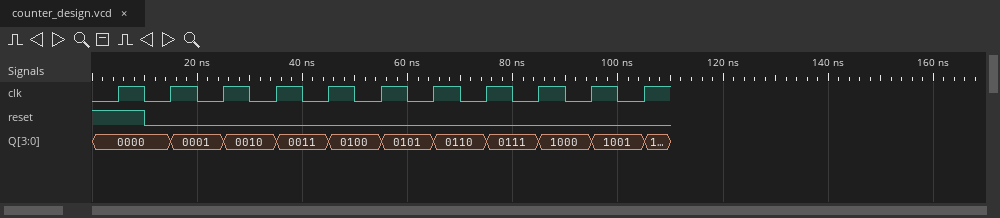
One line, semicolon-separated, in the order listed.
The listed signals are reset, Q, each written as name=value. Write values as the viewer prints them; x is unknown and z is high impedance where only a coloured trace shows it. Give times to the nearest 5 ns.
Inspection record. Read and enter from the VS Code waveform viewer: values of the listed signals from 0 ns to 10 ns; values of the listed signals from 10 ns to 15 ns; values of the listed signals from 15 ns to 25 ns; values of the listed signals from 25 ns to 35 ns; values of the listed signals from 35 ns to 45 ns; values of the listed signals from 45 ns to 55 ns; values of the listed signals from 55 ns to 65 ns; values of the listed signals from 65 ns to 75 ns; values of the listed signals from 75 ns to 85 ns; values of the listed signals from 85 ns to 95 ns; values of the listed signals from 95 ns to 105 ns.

reset=1, Q=0000; reset=0, Q=0000; reset=0, Q=0001; reset=0, Q=0010; reset=0, Q=0011; reset=0, Q=0100; reset=0, Q=0101; reset=0, Q=0110; reset=0, Q=0111; reset=0, Q=1000; reset=0, Q=1001
